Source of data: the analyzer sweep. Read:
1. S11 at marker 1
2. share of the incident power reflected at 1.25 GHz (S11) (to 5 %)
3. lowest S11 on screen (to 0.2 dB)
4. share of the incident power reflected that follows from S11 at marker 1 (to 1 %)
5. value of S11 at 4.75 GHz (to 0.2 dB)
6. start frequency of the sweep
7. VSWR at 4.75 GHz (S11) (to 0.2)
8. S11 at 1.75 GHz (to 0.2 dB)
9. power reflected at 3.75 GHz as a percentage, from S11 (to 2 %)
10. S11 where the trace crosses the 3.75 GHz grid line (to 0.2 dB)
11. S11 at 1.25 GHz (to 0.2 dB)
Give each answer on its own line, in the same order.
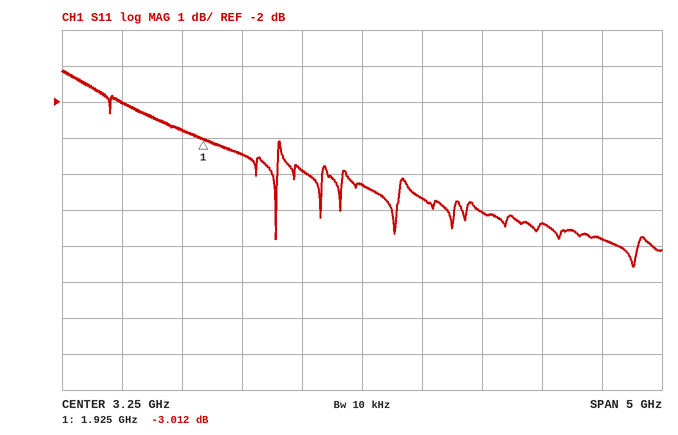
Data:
-3.012 dB
65 %
-6.6 dB
50 %
-5.4 dB
750 MHz
3.4
-2.8 dB
34 %
-4.6 dB
-2.0 dB
